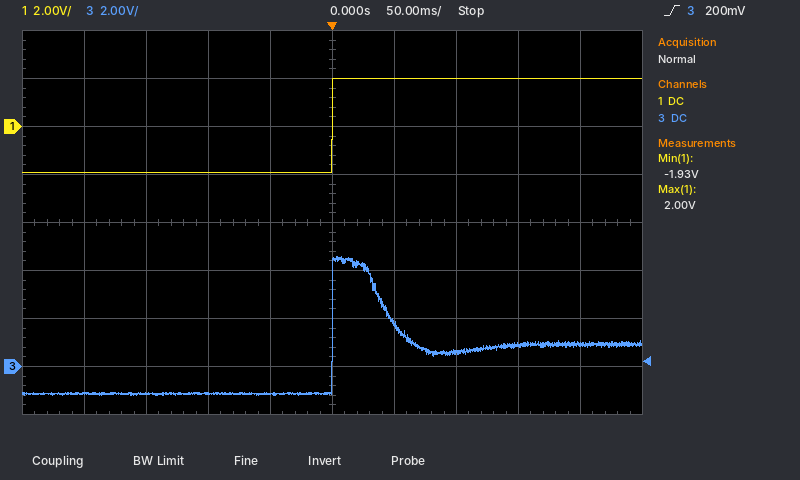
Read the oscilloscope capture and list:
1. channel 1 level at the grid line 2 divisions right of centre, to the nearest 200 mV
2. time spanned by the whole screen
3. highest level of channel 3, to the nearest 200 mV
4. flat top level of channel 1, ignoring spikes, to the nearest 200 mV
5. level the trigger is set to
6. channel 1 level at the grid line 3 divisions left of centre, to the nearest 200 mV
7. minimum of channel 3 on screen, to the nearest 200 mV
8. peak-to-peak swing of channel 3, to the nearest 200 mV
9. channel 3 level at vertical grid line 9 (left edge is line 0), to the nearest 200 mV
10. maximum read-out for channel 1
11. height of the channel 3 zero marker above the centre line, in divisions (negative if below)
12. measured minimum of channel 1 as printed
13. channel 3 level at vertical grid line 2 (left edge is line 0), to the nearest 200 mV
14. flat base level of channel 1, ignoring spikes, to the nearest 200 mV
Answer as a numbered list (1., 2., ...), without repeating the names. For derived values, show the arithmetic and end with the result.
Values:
1. 2.0 V
2. 500 ms
3. 4.6 V
4. 2.0 V
5. 200 mV
6. -2.0 V
7. -1.2 V
8. 4.6 V − (-1.2 V) = 5.8 V
9. 1.0 V
10. 2.00 V
11. -3.0 div
12. -1.93 V
13. -1.2 V
14. -2.0 V
